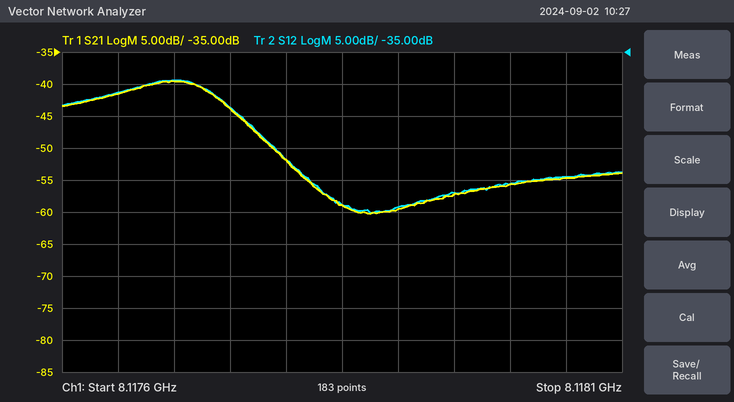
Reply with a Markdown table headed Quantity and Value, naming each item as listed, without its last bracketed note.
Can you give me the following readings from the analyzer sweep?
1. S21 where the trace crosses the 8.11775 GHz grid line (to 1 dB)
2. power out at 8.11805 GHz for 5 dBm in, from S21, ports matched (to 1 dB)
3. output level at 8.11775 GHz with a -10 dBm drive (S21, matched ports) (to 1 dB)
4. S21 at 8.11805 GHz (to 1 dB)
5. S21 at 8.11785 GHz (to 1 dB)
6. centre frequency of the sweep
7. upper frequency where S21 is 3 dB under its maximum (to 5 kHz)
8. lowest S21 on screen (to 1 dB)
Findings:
| Quantity | Value |
|---|---|
| S21 where the trace crosses the 8.11775 GHz grid line | -44 dB |
| power out at 8.11805 GHz for 5 dBm in, from S21, ports matched | -50 dBm |
| output level at 8.11775 GHz with a -10 dBm drive (S21, matched ports) | -54 dBm |
| S21 at 8.11805 GHz | -55 dB |
| S21 at 8.11785 GHz | -59 dB |
| centre frequency of the sweep | 8.11785 GHz |
| upper frequency where S21 is 3 dB under its maximum | 8.117740 GHz |
| lowest S21 on screen | -60 dB |
